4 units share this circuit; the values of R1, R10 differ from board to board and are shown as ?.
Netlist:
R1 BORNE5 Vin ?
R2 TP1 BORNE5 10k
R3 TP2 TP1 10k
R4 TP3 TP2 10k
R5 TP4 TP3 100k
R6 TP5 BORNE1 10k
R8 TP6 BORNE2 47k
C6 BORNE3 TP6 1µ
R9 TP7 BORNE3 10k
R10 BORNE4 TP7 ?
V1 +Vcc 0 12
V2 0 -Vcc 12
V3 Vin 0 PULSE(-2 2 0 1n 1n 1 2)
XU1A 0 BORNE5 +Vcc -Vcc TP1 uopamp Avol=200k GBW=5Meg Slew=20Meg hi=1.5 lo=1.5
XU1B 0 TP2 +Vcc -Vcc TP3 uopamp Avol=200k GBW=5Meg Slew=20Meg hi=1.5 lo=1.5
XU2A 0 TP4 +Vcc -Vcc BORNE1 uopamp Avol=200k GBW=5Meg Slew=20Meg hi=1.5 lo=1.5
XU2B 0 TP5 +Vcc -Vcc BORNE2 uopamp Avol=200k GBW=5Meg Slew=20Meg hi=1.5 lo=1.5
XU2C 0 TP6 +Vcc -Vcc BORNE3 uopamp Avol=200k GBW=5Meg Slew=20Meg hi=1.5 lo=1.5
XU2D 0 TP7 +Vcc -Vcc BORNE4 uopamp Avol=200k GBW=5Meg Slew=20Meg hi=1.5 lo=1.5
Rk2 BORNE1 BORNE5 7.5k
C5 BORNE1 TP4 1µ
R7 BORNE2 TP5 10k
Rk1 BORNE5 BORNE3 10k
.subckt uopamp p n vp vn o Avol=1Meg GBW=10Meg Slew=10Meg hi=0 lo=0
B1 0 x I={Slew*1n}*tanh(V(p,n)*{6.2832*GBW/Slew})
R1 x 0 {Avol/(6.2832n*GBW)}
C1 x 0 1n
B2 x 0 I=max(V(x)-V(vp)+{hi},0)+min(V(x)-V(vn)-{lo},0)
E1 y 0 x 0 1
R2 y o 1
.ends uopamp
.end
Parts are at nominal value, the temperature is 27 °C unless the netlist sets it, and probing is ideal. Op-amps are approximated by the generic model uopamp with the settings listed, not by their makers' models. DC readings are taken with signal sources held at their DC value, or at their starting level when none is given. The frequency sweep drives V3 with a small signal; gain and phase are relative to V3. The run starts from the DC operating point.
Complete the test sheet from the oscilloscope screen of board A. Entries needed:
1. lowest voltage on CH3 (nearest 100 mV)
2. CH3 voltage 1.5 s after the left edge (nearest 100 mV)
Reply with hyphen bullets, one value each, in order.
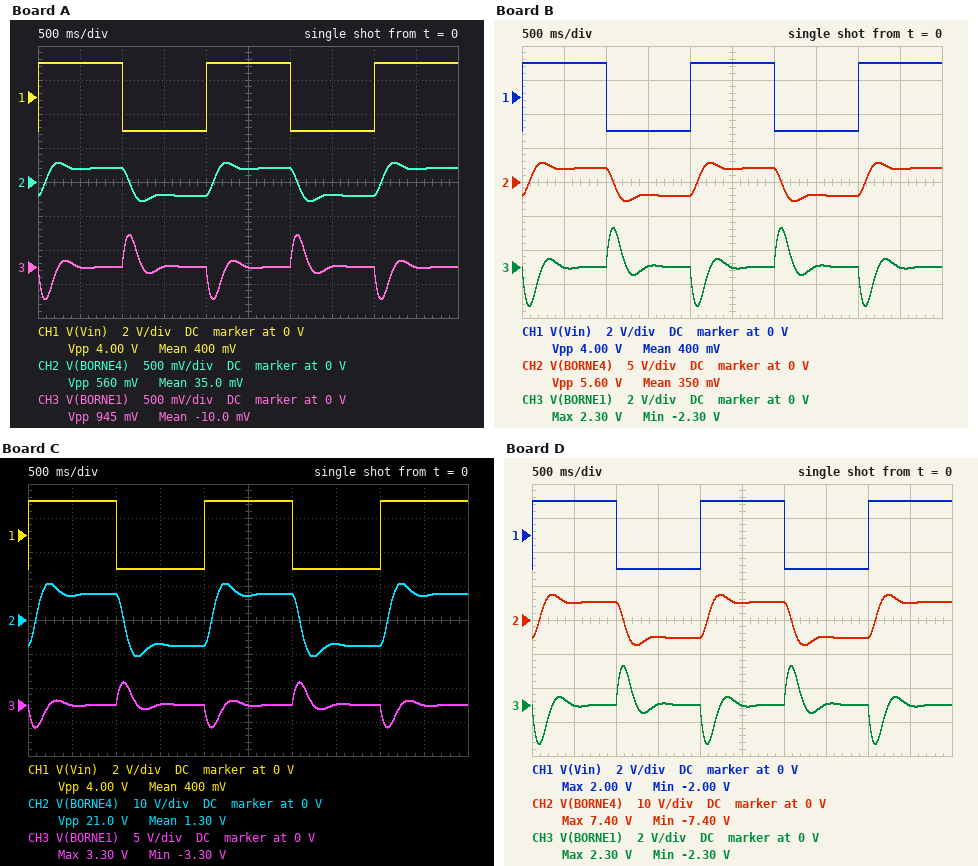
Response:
- -500 mV
- 0 V
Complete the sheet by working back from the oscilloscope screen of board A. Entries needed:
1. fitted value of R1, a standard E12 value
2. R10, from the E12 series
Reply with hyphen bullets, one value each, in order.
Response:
- 33 kΩ
- 3.3 kΩ
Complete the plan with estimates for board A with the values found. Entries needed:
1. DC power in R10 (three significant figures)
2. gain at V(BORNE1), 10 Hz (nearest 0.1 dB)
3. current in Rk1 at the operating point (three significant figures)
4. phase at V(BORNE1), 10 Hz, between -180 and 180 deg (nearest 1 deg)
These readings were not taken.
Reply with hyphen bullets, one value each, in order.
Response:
- 12.1 µW
- -26.1 dB
- 60.6 µA
- 103 deg
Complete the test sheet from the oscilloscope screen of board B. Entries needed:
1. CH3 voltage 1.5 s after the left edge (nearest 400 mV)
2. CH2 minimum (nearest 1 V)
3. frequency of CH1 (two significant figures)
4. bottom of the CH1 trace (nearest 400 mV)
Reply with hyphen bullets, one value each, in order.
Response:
- 0 V
- -3 V
- 500 mHz
- -2.0 V
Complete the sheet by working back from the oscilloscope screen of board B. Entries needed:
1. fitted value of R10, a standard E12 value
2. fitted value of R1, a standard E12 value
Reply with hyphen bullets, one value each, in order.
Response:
- 6.8 kΩ
- 6.8 kΩ
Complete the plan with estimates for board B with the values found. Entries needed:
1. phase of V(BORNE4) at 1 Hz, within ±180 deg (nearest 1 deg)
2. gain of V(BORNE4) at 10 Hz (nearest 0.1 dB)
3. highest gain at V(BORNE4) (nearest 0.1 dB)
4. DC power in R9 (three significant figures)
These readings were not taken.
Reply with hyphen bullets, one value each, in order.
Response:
- -26 deg
- -25.1 dB
- 1.8 dB
- 865 µW
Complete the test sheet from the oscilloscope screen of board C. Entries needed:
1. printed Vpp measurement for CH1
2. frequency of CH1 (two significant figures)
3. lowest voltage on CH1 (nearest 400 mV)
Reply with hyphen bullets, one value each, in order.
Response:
- 4.00 V
- 500 mHz
- -2.0 V
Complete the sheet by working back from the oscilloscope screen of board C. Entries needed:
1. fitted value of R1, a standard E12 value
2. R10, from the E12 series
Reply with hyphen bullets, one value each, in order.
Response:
- 4.7 kΩ
- 18 kΩ
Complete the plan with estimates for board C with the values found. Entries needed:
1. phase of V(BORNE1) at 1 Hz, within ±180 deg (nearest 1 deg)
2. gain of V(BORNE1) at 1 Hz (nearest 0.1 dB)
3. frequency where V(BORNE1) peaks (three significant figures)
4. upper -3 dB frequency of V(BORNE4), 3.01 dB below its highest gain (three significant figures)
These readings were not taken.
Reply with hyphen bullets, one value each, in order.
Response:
- -116 deg
- -3.2 dB
- 2.32 Hz
- 2.74 Hz
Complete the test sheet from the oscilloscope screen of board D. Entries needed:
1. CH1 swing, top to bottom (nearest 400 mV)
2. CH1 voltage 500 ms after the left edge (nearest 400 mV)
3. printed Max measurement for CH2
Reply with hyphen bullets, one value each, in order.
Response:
- 4.0 V
- 2.0 V
- 7.40 V
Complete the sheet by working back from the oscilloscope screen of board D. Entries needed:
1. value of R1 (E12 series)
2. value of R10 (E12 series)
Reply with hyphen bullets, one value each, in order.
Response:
- 6.8 kΩ
- 18 kΩ
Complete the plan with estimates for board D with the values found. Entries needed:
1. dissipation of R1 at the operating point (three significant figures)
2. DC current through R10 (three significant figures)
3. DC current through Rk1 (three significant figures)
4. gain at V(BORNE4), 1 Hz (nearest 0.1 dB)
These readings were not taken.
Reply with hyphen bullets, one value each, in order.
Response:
- 588 µW
- 294 µA
- 294 µA
- 9.3 dB
